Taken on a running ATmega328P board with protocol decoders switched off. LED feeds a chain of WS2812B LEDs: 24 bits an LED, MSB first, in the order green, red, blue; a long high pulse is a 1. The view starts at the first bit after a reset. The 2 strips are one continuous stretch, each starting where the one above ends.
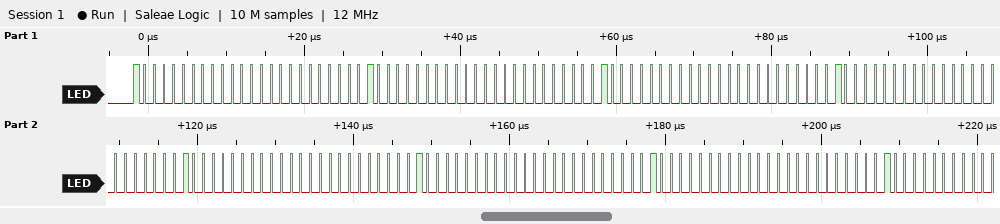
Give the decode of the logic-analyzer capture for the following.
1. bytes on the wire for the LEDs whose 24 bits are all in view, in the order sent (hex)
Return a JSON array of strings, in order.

["80 00 00 80 00 00 80 00 00 80 00 00 80 00 00 80 00 00 80 00 00"]
